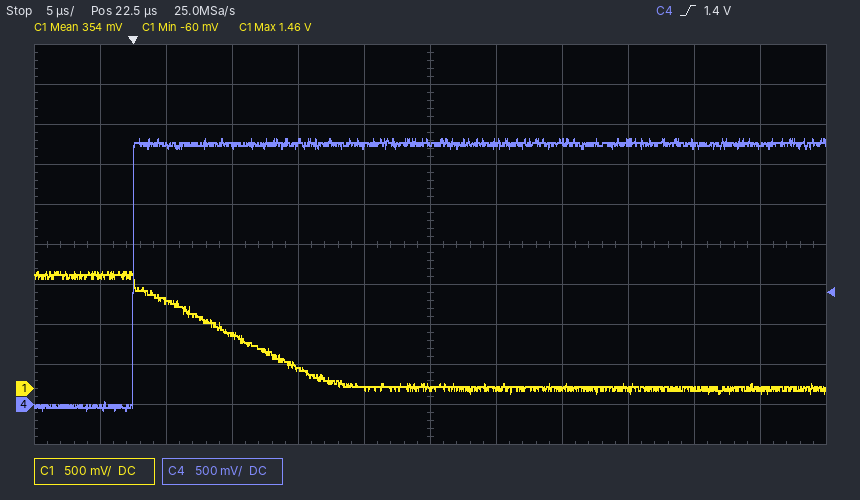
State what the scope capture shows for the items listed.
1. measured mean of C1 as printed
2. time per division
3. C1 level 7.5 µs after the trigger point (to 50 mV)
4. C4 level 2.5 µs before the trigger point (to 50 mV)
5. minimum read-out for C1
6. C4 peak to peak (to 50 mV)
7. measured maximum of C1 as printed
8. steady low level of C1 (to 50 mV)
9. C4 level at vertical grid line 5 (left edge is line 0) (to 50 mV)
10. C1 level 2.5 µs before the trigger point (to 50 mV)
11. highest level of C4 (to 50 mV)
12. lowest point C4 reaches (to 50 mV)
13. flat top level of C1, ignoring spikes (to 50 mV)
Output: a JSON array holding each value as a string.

["354 mV", "5 µs", "650 mV", "-50 mV", "-60 mV", "3.40 V", "1.46 V", "0 mV", "3.25 V", "1.40 V", "3.30 V", "-100 mV", "1.40 V"]
